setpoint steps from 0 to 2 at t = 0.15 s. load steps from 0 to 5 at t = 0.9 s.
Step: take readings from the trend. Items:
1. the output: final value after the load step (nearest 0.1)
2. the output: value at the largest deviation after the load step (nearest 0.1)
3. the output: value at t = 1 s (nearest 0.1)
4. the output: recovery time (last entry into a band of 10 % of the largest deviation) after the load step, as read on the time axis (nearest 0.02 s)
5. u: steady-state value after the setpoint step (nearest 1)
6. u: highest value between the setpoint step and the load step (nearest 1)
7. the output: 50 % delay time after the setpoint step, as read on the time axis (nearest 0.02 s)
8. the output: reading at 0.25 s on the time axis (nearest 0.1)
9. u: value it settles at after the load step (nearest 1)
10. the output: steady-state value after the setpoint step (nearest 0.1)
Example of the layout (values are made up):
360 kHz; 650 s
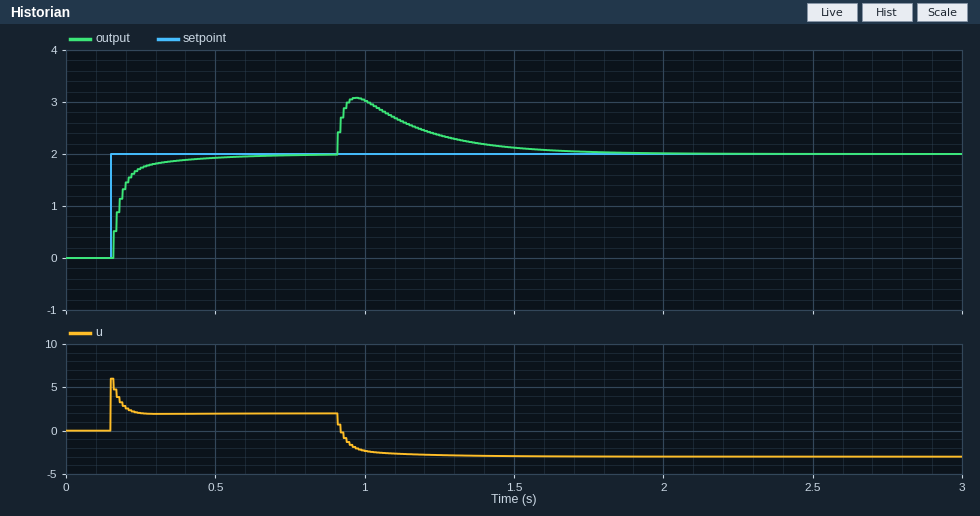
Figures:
2.0; 3.1; 3.0; 1.52 s; 2; 6; 0.18 s; 1.7; -3; 2.0
